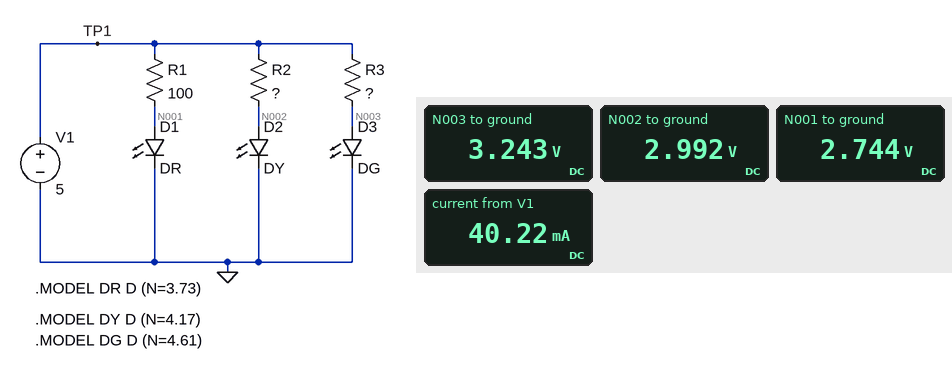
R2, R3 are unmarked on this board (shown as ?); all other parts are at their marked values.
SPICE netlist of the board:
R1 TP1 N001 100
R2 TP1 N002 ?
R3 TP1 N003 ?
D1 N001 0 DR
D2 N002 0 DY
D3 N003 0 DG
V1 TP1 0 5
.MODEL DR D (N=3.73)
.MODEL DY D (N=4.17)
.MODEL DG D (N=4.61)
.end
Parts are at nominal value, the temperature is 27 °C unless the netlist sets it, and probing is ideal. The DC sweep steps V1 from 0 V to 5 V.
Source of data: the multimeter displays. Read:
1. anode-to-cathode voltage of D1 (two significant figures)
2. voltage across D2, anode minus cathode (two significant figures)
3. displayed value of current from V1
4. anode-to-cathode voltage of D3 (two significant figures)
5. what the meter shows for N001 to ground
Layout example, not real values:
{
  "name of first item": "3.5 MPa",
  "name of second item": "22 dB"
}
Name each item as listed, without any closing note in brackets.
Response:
{
  "anode-to-cathode voltage of D1": "2.7 V",
  "voltage across D2, anode minus cathode": "3.0 V",
  "displayed value of current from V1": "40.22 mA",
  "anode-to-cathode voltage of D3": "3.2 V",
  "what the meter shows for N001 to ground": "2.744 V"
}
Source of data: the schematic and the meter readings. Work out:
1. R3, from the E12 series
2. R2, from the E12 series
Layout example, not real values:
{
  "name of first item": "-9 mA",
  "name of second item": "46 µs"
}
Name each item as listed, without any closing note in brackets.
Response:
{
  "R3, from the E12 series": "270 Ω",
  "R2, from the E12 series": "180 Ω"
}
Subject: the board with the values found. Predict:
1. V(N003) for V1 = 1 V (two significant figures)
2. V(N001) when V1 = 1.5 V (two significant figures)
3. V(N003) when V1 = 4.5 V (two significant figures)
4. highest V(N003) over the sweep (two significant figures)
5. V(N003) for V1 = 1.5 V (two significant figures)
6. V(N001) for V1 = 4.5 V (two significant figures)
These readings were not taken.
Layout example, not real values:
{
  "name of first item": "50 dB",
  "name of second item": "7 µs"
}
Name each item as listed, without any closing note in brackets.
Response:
{
  "V(N003) for V1 = 1 V": "1.0 V",
  "V(N001) when V1 = 1.5 V": "1.5 V",
  "V(N003) when V1 = 4.5 V": "3.2 V",
  "highest V(N003) over the sweep": "3.2 V",
  "V(N003) for V1 = 1.5 V": "1.5 V",
  "V(N001) for V1 = 4.5 V": "2.7 V"
}
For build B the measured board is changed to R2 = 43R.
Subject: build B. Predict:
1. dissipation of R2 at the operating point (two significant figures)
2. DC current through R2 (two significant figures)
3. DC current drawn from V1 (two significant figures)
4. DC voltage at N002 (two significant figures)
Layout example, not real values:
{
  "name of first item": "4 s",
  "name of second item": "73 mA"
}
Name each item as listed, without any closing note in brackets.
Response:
{
  "dissipation of R2 at the operating point": "81 mW",
  "DC current through R2": "43 mA",
  "DC current drawn from V1": "72 mA",
  "DC voltage at N002": "3.1 V"
}
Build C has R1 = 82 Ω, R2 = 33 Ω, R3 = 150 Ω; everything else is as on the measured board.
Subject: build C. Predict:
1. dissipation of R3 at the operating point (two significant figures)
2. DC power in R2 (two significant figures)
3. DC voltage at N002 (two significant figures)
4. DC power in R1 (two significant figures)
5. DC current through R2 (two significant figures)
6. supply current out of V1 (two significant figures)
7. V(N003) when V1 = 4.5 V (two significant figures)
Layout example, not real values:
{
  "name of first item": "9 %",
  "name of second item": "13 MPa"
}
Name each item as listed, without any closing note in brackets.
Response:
{
  "dissipation of R3 at the operating point": "19 mW",
  "DC power in R2": "100 mW",
  "DC voltage at N002": "3.2 V",
  "DC power in R1": "61 mW",
  "DC current through R2": "56 mA",
  "supply current out of V1": "94 mA",
  "V(N003) when V1 = 4.5 V": "3.3 V"
}
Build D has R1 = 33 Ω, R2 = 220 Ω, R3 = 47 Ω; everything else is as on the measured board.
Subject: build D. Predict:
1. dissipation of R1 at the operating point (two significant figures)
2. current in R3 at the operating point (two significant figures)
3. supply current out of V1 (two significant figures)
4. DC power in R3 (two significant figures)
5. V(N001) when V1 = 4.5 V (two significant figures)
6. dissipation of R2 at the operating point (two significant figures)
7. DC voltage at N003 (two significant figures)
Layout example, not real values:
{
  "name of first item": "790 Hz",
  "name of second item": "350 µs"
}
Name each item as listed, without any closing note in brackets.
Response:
{
  "dissipation of R1 at the operating point": "140 mW",
  "current in R3 at the operating point": "33 mA",
  "supply current out of V1": "110 mA",
  "DC power in R3": "52 mW",
  "V(N001) when V1 = 4.5 V": "2.8 V",
  "dissipation of R2 at the operating point": "19 mW",
  "DC voltage at N003": "3.4 V"
}
